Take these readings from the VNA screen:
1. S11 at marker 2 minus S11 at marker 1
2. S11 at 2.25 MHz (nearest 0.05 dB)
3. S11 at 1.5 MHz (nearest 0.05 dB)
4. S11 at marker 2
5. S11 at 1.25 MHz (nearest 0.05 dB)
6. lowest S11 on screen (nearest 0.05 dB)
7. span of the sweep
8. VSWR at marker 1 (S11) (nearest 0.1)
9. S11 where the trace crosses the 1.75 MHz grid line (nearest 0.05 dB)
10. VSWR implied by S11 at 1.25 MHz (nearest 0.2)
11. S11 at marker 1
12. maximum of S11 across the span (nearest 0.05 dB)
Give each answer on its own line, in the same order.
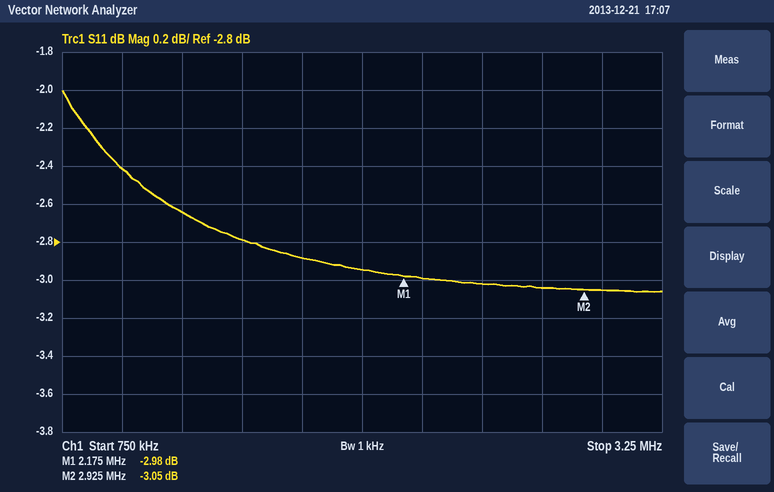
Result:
-0.07 dB
-3.00 dB
-2.80 dB
-3.05 dB
-2.65 dB
-3.05 dB
2.5 MHz
5.9
-2.90 dB
6.6
-2.98 dB
-2.00 dB
